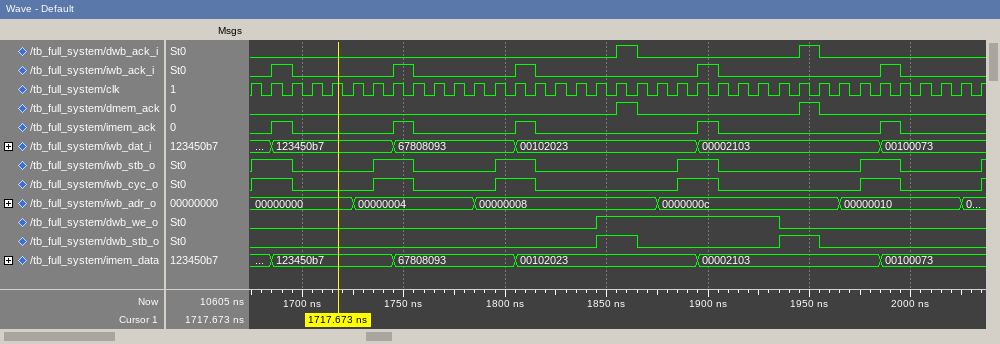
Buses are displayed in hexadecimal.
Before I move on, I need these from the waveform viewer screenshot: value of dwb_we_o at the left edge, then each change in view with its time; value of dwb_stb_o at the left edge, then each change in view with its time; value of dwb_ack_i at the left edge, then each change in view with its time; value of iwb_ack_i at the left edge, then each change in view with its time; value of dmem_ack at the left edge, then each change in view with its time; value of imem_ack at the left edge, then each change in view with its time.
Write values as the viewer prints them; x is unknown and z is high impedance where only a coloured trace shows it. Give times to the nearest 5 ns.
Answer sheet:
0, 1 at 1845 ns, 0 at 1935 ns
0, 1 at 1845 ns, 0 at 1865 ns, 1 at 1935 ns, 0 at 1955 ns
0, 1 at 1855 ns, 0 at 1865 ns, 1 at 1945 ns, 0 at 1955 ns
0, 1 at 1685 ns, 0 at 1695 ns, 1 at 1745 ns, 0 at 1755 ns, 1 at 1805 ns, 0 at 1815 ns, 1 at 1895 ns, 0 at 1905 ns, 1 at 1985 ns, 0 at 1995 ns
0, 1 at 1855 ns, 0 at 1865 ns, 1 at 1945 ns, 0 at 1955 ns
0, 1 at 1685 ns, 0 at 1695 ns, 1 at 1745 ns, 0 at 1755 ns, 1 at 1805 ns, 0 at 1815 ns, 1 at 1895 ns, 0 at 1905 ns, 1 at 1985 ns, 0 at 1995 ns
